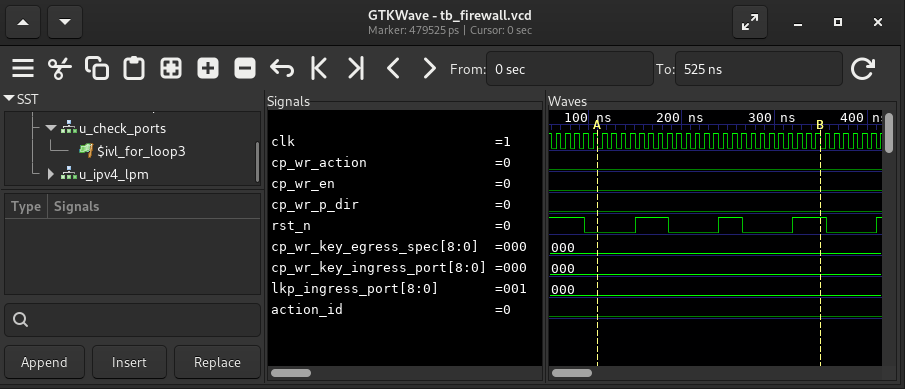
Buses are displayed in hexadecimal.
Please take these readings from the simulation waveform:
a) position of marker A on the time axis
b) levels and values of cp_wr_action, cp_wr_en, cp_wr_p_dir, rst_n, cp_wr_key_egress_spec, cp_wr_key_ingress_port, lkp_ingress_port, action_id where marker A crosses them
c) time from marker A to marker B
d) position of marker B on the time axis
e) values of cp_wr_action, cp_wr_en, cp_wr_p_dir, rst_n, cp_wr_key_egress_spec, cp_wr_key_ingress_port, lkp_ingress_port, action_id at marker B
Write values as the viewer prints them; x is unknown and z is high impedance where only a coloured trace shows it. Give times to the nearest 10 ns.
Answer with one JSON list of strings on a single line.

["110 ns", "cp_wr_action=0, cp_wr_en=0, cp_wr_p_dir=0, rst_n=0, cp_wr_key_egress_spec=000, cp_wr_key_ingress_port=000, lkp_ingress_port=000, action_id=0", "240 ns", "350 ns", "cp_wr_action=0, cp_wr_en=0, cp_wr_p_dir=0, rst_n=1, cp_wr_key_egress_spec=000, cp_wr_key_ingress_port=000, lkp_ingress_port=000, action_id=0"]
